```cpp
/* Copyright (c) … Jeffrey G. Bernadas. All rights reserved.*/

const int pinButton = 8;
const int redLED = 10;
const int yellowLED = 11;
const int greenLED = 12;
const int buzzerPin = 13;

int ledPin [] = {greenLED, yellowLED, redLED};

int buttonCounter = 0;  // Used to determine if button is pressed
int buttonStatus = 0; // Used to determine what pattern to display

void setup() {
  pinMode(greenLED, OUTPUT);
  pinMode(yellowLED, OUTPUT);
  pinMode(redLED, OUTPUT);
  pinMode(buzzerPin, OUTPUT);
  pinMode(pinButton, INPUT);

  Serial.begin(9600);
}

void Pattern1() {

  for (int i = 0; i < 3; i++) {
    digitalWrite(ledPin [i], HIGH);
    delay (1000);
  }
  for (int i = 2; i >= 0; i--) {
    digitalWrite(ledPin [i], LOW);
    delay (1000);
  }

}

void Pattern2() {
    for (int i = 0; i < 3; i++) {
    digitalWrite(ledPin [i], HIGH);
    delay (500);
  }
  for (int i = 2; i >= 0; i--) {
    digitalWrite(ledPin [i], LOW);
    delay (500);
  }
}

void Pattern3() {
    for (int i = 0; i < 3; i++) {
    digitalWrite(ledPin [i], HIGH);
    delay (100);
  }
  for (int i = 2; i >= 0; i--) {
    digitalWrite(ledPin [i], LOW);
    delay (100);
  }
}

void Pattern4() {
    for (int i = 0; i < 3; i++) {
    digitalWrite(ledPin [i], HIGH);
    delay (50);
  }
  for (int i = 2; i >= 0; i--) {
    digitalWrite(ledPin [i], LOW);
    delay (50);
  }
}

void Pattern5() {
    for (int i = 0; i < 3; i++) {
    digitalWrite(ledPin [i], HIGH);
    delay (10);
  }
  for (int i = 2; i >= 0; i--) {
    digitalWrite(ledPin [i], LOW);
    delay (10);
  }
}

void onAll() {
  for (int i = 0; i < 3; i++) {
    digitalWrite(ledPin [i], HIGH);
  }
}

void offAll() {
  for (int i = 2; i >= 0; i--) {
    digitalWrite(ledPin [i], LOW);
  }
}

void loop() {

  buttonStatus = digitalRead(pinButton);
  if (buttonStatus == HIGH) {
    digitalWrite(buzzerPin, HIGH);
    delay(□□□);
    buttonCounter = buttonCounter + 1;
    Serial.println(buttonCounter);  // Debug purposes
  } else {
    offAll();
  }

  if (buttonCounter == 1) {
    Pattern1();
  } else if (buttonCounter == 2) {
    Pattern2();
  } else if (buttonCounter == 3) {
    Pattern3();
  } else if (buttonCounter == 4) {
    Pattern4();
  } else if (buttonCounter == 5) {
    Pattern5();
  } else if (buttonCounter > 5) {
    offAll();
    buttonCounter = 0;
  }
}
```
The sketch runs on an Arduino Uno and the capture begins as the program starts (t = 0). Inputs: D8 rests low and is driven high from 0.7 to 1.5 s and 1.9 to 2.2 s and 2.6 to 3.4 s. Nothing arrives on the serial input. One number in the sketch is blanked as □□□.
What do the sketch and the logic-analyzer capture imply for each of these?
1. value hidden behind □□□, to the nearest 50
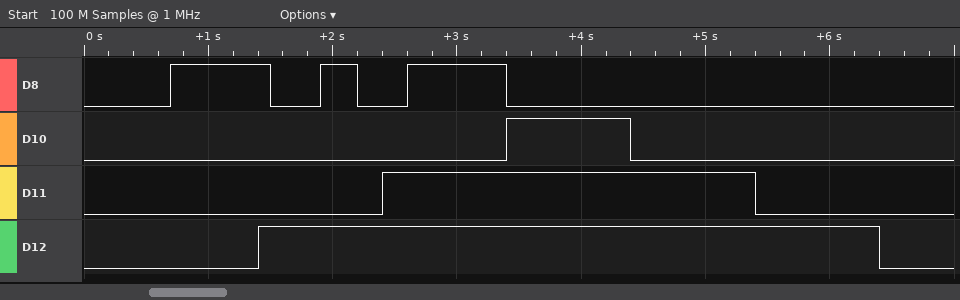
700
